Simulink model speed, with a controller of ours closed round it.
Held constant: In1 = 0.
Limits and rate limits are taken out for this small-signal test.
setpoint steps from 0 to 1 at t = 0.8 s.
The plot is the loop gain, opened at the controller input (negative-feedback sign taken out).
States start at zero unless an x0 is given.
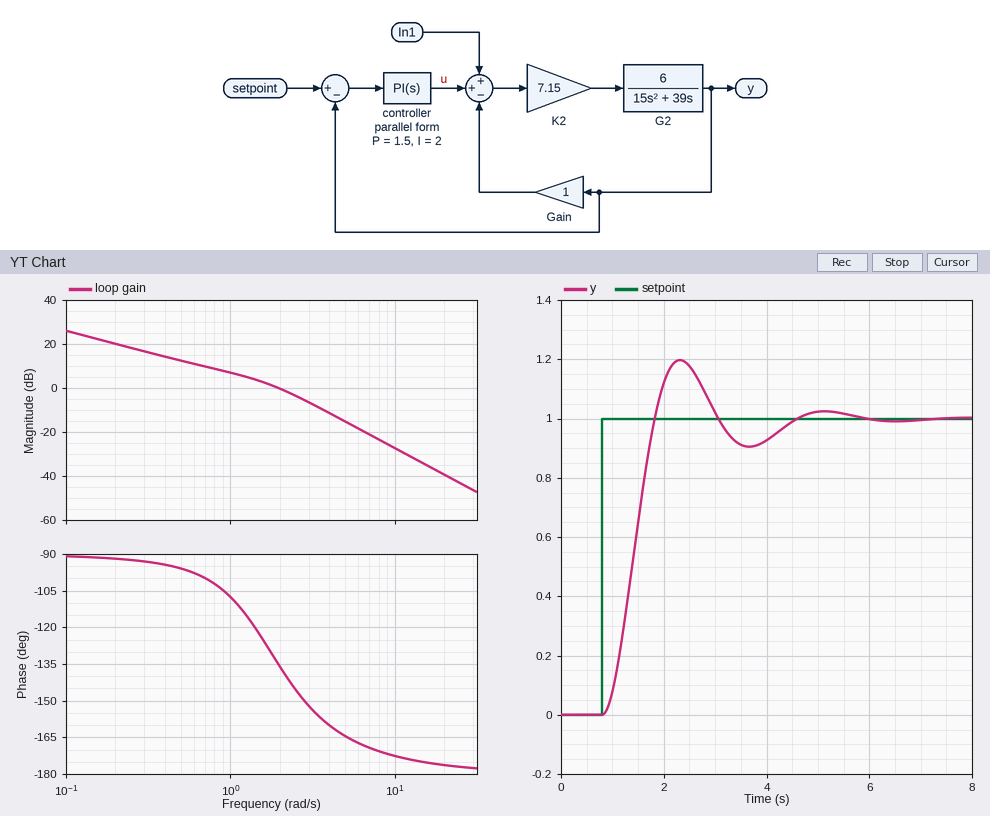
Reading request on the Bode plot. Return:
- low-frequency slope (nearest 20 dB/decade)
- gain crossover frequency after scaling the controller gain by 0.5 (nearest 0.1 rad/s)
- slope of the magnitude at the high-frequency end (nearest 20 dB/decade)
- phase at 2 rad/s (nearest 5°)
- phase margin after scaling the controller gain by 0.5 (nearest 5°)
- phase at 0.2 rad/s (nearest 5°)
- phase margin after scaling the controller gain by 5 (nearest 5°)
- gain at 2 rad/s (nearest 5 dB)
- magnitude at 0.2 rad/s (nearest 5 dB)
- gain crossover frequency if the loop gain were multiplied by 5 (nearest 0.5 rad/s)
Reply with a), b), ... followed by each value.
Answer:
a) -20 dB/decade
b) 1.1 rad/s
c) -40 dB/decade
d) -135°
e) 70°
f) -90°
g) 15°
h) 0 dB
i) 20 dB
j) 4.5 rad/s
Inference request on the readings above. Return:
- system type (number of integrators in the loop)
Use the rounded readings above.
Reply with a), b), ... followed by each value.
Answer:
a) 1
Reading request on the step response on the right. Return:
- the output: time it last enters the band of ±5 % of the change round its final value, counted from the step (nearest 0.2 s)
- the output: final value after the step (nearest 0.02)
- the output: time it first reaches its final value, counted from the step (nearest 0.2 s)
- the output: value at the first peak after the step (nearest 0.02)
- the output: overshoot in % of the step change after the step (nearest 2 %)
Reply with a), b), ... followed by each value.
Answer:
a) 3.4 s
b) 1.00
c) 1.0 s
d) 1.20
e) 20 %
